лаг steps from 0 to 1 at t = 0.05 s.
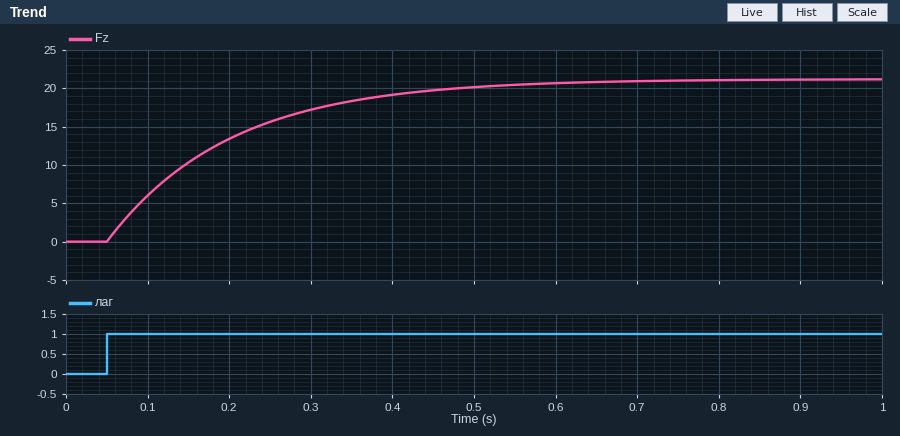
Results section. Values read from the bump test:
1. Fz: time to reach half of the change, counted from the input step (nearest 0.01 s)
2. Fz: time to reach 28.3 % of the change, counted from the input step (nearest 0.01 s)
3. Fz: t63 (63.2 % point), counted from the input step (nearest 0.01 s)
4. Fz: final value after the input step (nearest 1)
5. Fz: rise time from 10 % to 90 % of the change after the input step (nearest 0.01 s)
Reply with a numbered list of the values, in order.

1. 0.10 s
2. 0.05 s
3. 0.15 s
4. 21
5. 0.33 s
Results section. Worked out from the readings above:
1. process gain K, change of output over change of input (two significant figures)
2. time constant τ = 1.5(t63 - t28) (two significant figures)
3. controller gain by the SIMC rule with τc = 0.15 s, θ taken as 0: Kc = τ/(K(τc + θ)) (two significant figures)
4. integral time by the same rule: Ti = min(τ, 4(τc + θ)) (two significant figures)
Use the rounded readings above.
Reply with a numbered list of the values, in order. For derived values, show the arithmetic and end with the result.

1. (21 - 0) / 1 = 21
2. 1.5 × (0.15 - 0.05) = 0.15 s
3. 0.15 / (21 × (0.15 + 0)) = 0.048
4. min(0.15, 4 × (0.15 + 0)) = 0.15 s
